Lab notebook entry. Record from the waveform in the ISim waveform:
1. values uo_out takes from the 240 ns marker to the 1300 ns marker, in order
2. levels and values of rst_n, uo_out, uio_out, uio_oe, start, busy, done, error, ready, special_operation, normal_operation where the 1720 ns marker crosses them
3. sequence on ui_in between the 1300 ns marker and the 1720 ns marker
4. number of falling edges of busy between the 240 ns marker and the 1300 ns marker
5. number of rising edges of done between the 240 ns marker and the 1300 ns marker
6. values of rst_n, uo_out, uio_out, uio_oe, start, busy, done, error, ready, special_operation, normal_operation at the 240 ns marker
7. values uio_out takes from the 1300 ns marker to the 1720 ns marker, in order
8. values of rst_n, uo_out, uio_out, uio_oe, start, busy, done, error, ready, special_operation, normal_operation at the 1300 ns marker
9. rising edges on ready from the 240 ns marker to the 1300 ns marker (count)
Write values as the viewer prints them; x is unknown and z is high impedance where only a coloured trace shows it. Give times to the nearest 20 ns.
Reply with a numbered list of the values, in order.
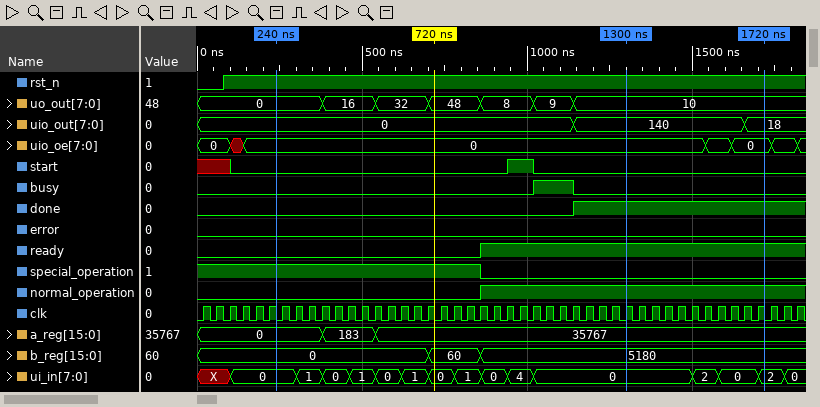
1. 0, 16, 32, 48, 8, 9, 10
2. rst_n=1, uo_out=10, uio_out=18, uio_oe=0, start=0, busy=0, done=1, error=0, ready=1, special_operation=0, normal_operation=1
3. 0, 2, 0, 2
4. 1
5. 1
6. rst_n=1, uo_out=0, uio_out=0, uio_oe=0, start=0, busy=0, done=0, error=0, ready=0, special_operation=1, normal_operation=0
7. 140, 18
8. rst_n=1, uo_out=10, uio_out=140, uio_oe=0, start=0, busy=0, done=1, error=0, ready=1, special_operation=0, normal_operation=1
9. 1
